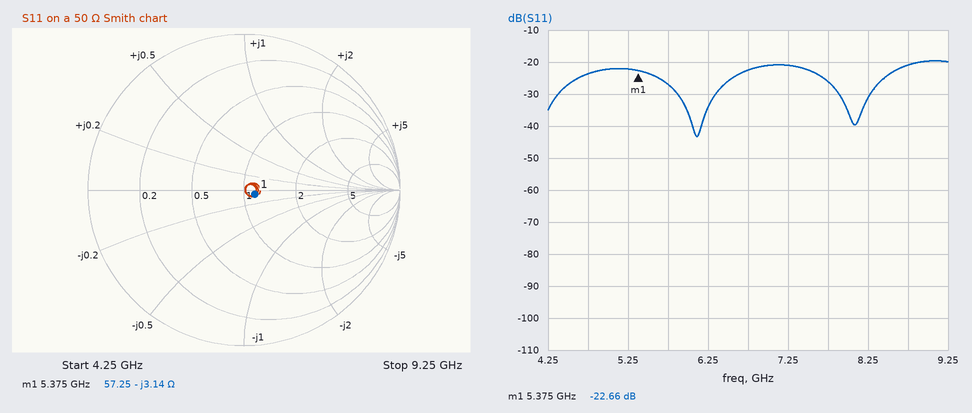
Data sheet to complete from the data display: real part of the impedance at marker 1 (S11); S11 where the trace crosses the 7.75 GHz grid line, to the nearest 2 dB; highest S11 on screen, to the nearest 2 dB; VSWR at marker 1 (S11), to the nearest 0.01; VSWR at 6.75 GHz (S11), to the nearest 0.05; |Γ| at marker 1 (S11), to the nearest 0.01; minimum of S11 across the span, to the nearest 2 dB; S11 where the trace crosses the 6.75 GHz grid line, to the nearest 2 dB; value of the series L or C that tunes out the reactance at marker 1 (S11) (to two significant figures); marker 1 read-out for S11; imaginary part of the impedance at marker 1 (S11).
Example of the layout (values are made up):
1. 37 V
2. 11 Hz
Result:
1. 57.25 Ω
2. -26 dB
3. -20 dB
4. 1.16
5. 1.15
6. 0.07
7. -44 dB
8. -22 dB
9. 93 pH
10. -22.66 dB
11. -3.14 Ω
